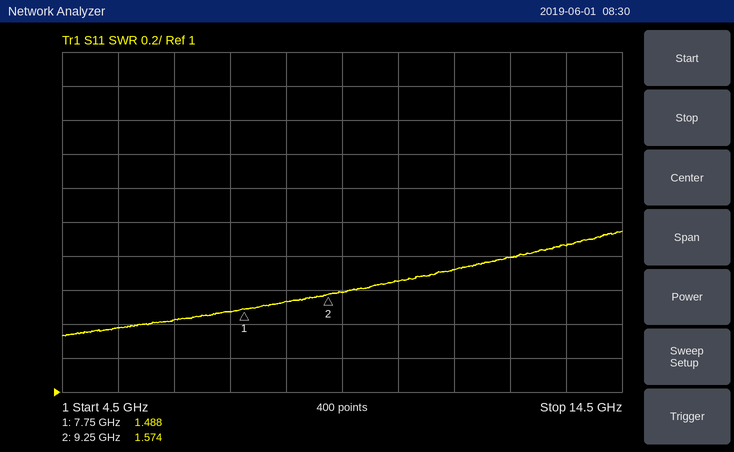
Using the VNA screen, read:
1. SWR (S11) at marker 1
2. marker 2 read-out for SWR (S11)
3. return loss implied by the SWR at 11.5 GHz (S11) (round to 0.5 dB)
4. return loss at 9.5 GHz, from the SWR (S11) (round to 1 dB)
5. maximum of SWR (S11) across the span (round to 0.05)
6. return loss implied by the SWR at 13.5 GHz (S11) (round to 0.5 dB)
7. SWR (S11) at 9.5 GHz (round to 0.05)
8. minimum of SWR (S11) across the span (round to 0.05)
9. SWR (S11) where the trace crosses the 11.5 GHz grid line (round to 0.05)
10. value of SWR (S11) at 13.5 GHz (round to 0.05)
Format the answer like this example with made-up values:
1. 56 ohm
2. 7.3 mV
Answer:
1. 1.488
2. 1.574
3. 11.5 dB
4. 13 dB
5. 1.95
6. 10.5 dB
7. 1.60
8. 1.35
9. 1.70
10. 1.85
